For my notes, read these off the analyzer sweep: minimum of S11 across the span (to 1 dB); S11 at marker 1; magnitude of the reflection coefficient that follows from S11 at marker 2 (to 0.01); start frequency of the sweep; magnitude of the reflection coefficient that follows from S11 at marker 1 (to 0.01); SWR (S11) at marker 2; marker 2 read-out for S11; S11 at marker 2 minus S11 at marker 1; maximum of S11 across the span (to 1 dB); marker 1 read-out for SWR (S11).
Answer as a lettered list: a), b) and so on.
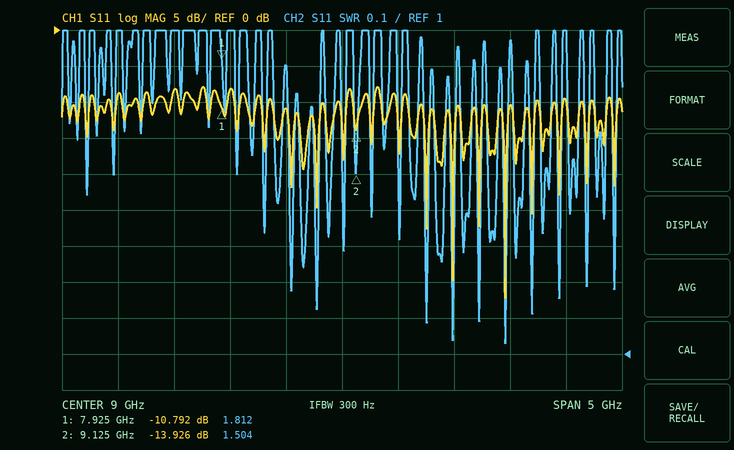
a) -37 dB
b) -10.792 dB
c) 0.20
d) 6.5 GHz
e) 0.29
f) 1.504
g) -13.926 dB
h) -3.134 dB
i) -8 dB
j) 1.812
